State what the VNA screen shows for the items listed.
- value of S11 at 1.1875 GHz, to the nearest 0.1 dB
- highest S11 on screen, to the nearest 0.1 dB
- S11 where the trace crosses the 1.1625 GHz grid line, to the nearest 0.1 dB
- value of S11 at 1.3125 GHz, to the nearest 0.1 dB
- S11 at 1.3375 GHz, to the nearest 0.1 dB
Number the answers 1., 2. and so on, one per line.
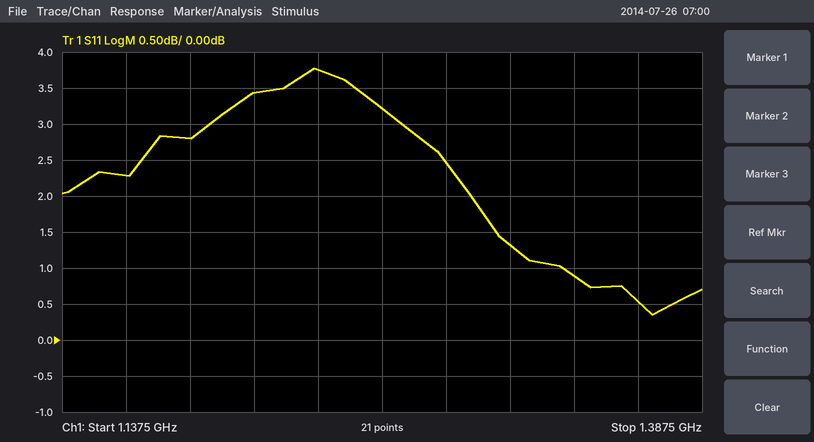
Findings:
1. 2.8 dB
2. 3.8 dB
3. 2.3 dB
4. 1.3 dB
5. 0.9 dB
